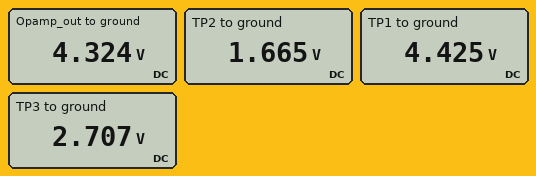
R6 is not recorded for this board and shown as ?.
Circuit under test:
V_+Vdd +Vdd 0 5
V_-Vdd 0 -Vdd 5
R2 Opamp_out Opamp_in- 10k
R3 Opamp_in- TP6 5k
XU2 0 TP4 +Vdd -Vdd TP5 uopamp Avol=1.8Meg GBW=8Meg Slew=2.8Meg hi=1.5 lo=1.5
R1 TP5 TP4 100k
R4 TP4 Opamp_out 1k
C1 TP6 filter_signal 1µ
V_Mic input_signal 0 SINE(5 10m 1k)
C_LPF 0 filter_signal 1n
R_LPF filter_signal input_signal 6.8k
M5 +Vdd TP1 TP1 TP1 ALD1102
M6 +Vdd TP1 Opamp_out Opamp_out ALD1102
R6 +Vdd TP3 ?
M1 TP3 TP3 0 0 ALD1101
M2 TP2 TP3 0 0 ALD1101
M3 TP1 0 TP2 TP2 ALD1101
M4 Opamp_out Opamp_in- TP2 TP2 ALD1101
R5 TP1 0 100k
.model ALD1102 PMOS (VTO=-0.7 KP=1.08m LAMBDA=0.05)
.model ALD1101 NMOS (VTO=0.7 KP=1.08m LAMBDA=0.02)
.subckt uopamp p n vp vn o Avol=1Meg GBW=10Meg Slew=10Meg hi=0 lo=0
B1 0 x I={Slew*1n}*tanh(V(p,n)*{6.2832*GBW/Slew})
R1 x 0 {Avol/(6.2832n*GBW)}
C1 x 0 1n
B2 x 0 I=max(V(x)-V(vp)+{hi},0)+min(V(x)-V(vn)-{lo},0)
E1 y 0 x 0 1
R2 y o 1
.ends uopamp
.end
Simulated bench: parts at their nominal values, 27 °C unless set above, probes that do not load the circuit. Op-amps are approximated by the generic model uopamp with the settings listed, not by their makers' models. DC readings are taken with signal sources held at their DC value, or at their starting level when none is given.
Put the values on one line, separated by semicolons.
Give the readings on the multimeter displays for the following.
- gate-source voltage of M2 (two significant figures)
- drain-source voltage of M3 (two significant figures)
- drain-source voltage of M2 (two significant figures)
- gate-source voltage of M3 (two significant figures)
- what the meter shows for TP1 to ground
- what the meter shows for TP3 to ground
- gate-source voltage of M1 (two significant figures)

2.7 V; 2.8 V; 1.7 V; -1.7 V; 4.425 V; 2.707 V; 2.7 V
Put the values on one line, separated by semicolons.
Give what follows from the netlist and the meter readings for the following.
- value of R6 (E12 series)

1 kΩ
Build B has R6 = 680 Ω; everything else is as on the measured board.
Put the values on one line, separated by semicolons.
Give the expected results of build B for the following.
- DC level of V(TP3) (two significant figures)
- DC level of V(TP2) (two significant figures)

3.0 V; 1.5 V
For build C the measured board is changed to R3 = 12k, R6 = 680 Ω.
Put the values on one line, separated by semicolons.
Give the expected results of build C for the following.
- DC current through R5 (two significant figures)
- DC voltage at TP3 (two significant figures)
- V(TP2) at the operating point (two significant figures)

44 µA; 3.0 V; 1.5 V
